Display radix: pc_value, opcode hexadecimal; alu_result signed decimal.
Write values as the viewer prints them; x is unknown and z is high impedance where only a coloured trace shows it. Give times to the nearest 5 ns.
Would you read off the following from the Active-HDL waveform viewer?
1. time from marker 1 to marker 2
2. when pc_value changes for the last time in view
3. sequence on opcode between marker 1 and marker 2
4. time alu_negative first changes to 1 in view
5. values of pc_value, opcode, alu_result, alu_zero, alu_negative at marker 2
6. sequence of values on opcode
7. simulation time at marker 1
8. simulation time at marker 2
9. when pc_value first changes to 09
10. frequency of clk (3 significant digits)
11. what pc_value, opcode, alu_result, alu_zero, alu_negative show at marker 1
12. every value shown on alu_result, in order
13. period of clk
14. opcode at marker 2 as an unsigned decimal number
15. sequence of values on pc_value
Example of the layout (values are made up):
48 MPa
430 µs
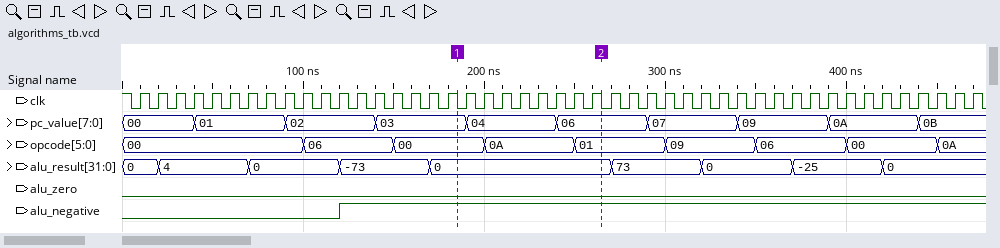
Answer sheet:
80 ns
440 ns
00, 0A, 01
120 ns
pc_value=06, opcode=01, alu_result=0, alu_zero=0, alu_negative=1
00, 06, 00, 0A, 01, 09, 06, 00, 0A
185 ns
265 ns
340 ns
100 MHz
pc_value=03, opcode=00, alu_result=0, alu_zero=0, alu_negative=1
0, 4, 0, -73, 0, 73, 0, -25, 0
10 ns
1
00, 01, 02, 03, 04, 06, 07, 09, 0A, 0B
